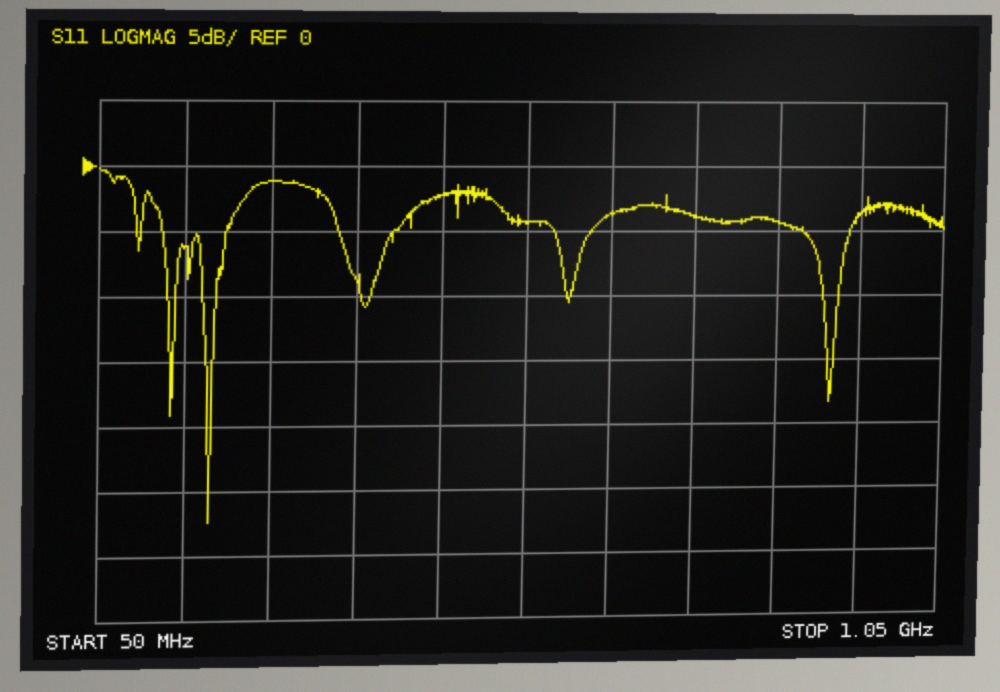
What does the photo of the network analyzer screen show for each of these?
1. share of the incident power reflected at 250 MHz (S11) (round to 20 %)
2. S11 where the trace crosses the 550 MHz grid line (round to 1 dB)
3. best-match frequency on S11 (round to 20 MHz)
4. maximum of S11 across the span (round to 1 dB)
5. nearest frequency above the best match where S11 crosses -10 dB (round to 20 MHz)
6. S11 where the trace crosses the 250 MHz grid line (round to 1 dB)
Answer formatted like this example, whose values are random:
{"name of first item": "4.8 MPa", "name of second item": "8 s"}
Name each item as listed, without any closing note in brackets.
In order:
{"share of the incident power reflected at 250 MHz (S11)": "80 %", "S11 where the trace crosses the 550 MHz grid line": "-4 dB", "best-match frequency on S11": "180 MHz", "maximum of S11 across the span": "0 dB", "nearest frequency above the best match where S11 crosses -10 dB": "180 MHz", "S11 where the trace crosses the 250 MHz grid line": "-1 dB"}
